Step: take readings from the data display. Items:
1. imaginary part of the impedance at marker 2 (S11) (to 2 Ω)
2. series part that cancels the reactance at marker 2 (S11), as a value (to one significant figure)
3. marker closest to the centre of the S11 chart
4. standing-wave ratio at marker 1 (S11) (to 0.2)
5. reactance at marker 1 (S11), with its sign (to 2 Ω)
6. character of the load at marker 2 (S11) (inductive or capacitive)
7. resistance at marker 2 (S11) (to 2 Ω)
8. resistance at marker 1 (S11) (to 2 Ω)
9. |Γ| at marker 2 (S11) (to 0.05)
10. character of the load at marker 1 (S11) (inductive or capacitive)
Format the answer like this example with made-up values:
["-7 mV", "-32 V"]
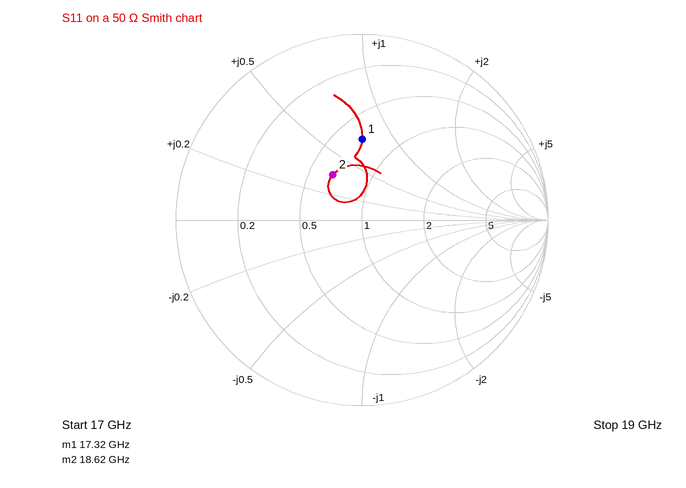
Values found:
["+18 Ω", "500 fF", "marker 2", "2.6", "+36 Ω", "inductive", "32 Ω", "34 Ω", "0.30", "inductive"]
